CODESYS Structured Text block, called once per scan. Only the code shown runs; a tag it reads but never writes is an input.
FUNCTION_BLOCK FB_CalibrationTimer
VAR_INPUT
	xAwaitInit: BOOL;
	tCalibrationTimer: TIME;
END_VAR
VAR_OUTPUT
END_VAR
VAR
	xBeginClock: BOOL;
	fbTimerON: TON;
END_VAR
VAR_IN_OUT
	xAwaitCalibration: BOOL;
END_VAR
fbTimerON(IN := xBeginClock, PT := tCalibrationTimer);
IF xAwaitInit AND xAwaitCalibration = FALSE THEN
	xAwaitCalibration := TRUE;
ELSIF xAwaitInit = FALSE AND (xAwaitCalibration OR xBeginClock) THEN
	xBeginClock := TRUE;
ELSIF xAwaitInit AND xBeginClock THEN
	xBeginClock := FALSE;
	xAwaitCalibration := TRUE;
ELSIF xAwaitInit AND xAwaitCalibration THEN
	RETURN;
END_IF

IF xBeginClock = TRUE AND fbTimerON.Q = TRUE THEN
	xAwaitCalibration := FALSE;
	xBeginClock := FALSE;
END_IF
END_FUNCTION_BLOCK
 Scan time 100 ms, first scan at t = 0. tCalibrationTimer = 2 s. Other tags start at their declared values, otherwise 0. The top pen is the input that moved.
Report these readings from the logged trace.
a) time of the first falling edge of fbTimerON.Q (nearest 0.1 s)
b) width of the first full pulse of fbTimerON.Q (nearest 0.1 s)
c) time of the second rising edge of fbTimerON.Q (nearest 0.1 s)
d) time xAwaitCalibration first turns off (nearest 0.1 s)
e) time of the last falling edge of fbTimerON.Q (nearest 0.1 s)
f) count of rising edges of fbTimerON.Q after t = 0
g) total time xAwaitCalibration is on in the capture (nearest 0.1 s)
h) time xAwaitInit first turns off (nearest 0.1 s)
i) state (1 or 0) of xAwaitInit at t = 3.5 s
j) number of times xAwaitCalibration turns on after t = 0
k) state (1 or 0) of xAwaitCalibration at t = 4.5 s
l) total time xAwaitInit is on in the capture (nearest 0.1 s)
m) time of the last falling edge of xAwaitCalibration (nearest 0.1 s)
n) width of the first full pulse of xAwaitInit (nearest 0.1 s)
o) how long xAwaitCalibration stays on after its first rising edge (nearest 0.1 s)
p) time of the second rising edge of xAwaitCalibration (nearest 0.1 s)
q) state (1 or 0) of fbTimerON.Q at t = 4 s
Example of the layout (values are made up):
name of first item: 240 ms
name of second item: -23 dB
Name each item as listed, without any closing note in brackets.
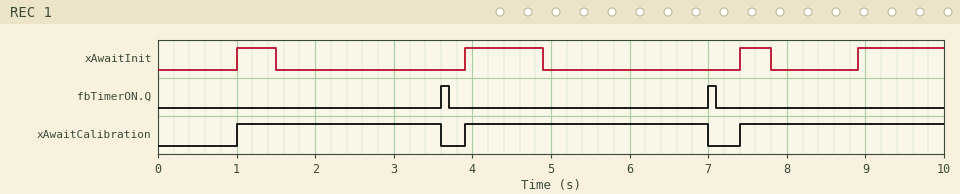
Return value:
time of the first falling edge of fbTimerON.Q: 3.7 s
width of the first full pulse of fbTimerON.Q: 0.1 s
time of the second rising edge of fbTimerON.Q: 7.0 s
time xAwaitCalibration first turns off: 3.6 s
time of the last falling edge of fbTimerON.Q: 7.1 s
count of rising edges of fbTimerON.Q after t = 0: 2
total time xAwaitCalibration is on in the capture: 8.3 s
time xAwaitInit first turns off: 1.5 s
state (1 or 0) of xAwaitInit at t = 3.5 s: 0
number of times xAwaitCalibration turns on after t = 0: 3
state (1 or 0) of xAwaitCalibration at t = 4.5 s: 1
total time xAwaitInit is on in the capture: 3.0 s
time of the last falling edge of xAwaitCalibration: 7.0 s
width of the first full pulse of xAwaitInit: 0.5 s
how long xAwaitCalibration stays on after its first rising edge: 2.6 s
time of the second rising edge of xAwaitCalibration: 3.9 s
state (1 or 0) of fbTimerON.Q at t = 4 s: 0
